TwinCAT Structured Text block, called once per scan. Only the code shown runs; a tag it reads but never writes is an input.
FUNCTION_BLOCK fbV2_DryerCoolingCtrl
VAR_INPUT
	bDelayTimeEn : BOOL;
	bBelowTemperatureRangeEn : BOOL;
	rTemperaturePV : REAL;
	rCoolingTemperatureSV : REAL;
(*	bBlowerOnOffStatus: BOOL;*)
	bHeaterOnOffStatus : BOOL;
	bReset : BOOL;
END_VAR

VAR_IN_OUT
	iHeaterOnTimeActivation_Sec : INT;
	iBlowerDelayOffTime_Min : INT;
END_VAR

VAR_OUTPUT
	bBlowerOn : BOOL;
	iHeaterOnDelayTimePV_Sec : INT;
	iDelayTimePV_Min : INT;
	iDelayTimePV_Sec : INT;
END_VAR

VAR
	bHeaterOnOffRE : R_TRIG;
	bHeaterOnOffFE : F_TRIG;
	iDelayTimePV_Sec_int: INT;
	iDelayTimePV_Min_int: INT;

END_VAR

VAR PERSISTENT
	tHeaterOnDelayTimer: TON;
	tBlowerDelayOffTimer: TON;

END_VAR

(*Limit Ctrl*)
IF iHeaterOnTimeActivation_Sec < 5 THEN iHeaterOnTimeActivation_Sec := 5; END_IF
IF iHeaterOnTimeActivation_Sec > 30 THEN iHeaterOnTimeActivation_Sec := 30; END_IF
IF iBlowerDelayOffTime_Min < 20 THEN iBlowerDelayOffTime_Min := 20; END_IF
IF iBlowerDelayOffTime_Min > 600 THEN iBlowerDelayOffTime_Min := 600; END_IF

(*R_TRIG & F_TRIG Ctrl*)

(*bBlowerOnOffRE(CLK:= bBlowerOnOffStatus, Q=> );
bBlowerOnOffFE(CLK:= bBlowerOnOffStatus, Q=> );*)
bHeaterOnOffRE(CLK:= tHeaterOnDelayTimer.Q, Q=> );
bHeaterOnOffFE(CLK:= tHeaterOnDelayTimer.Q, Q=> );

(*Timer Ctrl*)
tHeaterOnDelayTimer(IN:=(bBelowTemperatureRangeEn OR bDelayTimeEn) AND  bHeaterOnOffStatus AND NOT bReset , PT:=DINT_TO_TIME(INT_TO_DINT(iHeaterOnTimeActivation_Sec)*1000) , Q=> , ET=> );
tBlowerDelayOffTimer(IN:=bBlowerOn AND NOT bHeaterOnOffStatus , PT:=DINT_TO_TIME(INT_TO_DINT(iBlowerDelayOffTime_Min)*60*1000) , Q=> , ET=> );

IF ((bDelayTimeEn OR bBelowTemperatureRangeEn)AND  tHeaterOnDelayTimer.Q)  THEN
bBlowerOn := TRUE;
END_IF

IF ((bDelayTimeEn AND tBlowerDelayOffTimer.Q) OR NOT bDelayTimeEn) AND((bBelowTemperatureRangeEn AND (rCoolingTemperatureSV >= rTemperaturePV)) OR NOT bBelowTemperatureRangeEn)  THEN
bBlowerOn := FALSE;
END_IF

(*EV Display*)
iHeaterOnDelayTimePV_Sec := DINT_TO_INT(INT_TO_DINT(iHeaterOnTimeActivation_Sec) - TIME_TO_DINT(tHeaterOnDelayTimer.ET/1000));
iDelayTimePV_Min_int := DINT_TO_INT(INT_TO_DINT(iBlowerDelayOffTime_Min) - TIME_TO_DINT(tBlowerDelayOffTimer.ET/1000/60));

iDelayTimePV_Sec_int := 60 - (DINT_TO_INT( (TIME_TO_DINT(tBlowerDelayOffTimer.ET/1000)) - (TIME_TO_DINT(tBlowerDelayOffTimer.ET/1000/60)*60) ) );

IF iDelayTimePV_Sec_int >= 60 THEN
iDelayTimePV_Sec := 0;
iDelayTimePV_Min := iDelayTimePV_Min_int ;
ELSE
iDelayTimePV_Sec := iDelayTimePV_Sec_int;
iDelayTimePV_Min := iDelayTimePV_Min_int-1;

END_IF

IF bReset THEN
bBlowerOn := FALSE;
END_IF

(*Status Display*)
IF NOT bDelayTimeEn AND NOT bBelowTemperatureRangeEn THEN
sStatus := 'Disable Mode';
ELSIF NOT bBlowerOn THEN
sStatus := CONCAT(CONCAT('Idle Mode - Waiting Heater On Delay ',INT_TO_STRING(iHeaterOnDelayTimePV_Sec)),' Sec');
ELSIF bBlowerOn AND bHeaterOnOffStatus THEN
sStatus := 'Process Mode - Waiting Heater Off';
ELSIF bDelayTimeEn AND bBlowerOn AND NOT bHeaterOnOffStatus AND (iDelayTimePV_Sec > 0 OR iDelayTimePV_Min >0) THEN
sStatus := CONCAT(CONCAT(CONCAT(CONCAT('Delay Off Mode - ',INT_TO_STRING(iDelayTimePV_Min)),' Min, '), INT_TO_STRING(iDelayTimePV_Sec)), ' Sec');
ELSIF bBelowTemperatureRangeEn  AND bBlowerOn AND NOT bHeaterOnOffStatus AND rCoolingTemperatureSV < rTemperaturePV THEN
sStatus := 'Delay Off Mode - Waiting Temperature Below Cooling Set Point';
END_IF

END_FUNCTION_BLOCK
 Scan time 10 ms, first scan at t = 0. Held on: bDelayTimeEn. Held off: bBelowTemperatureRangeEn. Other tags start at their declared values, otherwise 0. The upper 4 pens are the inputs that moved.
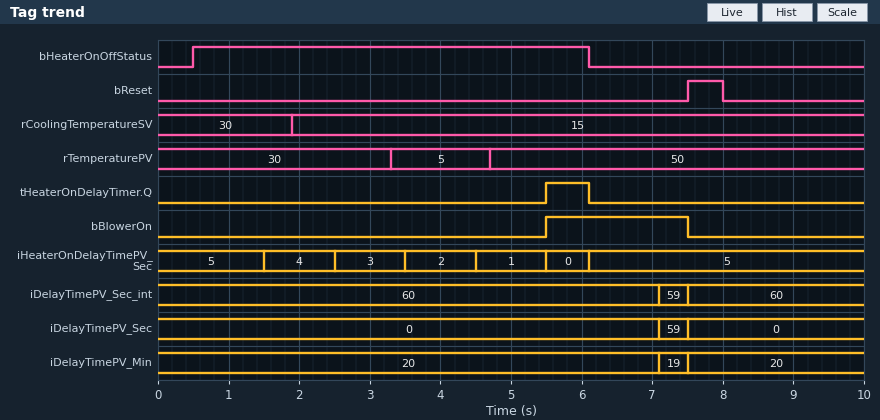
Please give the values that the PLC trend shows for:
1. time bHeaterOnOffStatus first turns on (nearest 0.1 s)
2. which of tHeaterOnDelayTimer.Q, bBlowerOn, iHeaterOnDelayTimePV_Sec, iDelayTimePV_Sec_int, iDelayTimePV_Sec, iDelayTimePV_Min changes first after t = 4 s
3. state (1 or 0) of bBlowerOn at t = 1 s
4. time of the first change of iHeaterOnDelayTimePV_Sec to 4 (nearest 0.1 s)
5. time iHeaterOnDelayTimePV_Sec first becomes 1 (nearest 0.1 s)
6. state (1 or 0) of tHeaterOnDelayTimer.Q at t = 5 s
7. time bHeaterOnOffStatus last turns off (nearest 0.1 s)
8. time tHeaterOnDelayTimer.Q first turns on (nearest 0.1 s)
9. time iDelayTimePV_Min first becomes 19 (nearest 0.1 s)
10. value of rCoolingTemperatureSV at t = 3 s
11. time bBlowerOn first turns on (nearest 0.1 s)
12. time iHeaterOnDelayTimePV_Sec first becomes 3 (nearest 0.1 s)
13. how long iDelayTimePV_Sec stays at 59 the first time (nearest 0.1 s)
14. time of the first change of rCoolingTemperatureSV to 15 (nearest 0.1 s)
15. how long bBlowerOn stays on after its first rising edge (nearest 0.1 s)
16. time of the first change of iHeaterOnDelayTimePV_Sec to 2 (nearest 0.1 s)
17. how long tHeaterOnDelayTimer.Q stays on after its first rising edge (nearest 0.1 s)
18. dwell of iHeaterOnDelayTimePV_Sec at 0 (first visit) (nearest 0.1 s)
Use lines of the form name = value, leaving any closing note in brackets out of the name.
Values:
time bHeaterOnOffStatus first turns on = 0.5 s
which of tHeaterOnDelayTimer.Q, bBlowerOn, iHeaterOnDelayTimePV_Sec, iDelayTimePV_Sec_int, iDelayTimePV_Sec, iDelayTimePV_Min changes first after t = 4 s = iHeaterOnDelayTimePV_Sec
state (1 or 0) of bBlowerOn at t = 1 s = 0
time of the first change of iHeaterOnDelayTimePV_Sec to 4 = 1.5 s
time iHeaterOnDelayTimePV_Sec first becomes 1 = 4.5 s
state (1 or 0) of tHeaterOnDelayTimer.Q at t = 5 s = 0
time bHeaterOnOffStatus last turns off = 6.1 s
time tHeaterOnDelayTimer.Q first turns on = 5.5 s
time iDelayTimePV_Min first becomes 19 = 7.1 s
value of rCoolingTemperatureSV at t = 3 s = 15
time bBlowerOn first turns on = 5.5 s
time iHeaterOnDelayTimePV_Sec first becomes 3 = 2.5 s
how long iDelayTimePV_Sec stays at 59 the first time = 0.4 s
time of the first change of rCoolingTemperatureSV to 15 = 1.9 s
how long bBlowerOn stays on after its first rising edge = 2.0 s
time of the first change of iHeaterOnDelayTimePV_Sec to 2 = 3.5 s
how long tHeaterOnDelayTimer.Q stays on after its first rising edge = 0.6 s
dwell of iHeaterOnDelayTimePV_Sec at 0 (first visit) = 0.6 s
